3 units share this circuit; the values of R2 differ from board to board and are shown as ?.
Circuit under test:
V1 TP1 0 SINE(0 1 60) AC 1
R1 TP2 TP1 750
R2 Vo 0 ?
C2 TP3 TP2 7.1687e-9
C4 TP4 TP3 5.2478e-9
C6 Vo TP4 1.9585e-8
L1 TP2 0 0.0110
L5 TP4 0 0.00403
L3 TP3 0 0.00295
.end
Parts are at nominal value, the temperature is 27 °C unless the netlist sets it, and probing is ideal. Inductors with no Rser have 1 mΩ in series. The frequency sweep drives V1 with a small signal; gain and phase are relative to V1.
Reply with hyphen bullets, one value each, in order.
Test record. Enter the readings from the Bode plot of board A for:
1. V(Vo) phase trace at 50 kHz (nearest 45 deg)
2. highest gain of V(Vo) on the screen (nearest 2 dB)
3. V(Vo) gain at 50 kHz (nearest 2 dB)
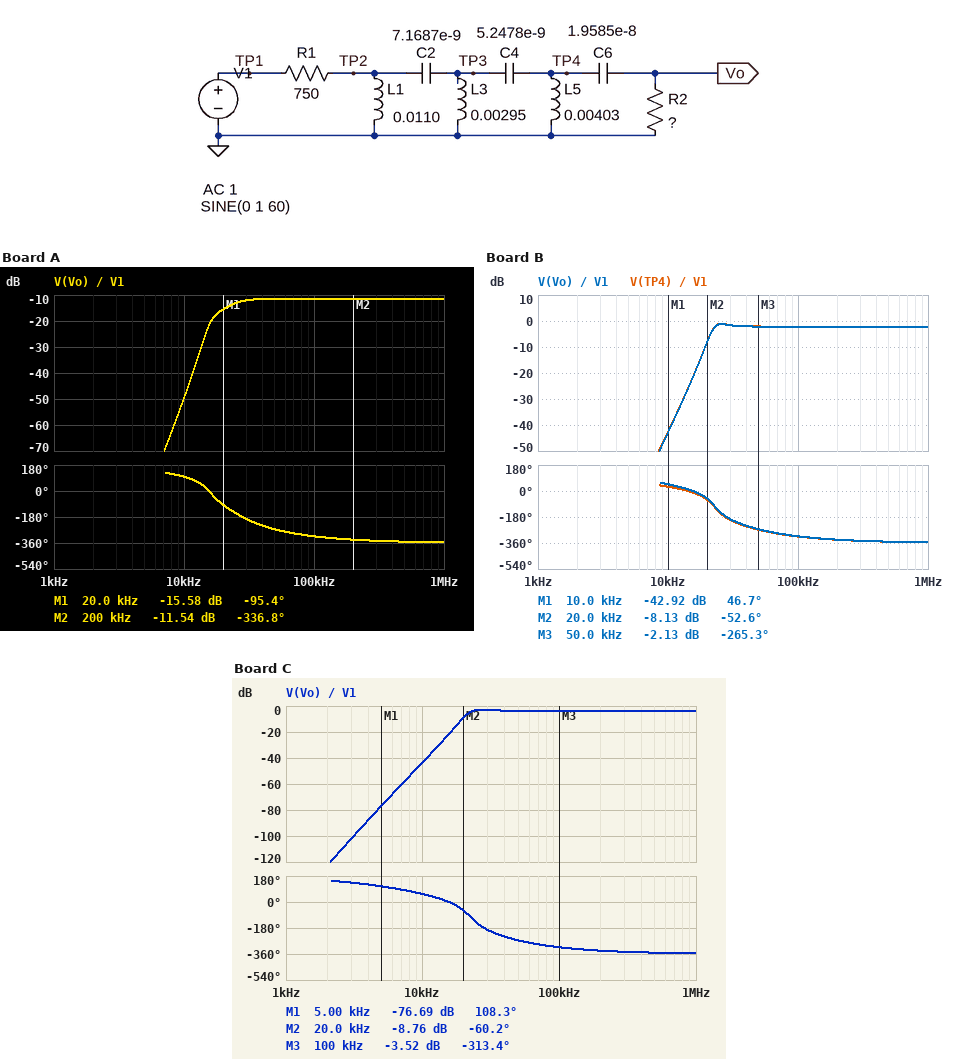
- -270 deg
- -12 dB
- -12 dB
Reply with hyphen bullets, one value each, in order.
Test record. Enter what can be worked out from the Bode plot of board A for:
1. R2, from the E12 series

- 270 Ω
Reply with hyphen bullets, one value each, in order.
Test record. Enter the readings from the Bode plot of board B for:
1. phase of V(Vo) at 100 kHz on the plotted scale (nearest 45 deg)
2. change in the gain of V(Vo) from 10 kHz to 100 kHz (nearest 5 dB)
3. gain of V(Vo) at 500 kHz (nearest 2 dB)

- -315 deg
- 40 dB
- -2 dB
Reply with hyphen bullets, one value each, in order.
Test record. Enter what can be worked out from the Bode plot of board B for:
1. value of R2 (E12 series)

- 2.7 kΩ
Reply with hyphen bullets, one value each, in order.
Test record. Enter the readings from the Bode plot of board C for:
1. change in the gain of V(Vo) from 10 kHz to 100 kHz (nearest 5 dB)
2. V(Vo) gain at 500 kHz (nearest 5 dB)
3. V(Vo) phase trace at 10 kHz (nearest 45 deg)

- 40 dB
- -5 dB
- 45 deg
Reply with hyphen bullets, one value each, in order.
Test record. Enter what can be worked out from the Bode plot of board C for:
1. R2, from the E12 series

- 1.5 kΩ
